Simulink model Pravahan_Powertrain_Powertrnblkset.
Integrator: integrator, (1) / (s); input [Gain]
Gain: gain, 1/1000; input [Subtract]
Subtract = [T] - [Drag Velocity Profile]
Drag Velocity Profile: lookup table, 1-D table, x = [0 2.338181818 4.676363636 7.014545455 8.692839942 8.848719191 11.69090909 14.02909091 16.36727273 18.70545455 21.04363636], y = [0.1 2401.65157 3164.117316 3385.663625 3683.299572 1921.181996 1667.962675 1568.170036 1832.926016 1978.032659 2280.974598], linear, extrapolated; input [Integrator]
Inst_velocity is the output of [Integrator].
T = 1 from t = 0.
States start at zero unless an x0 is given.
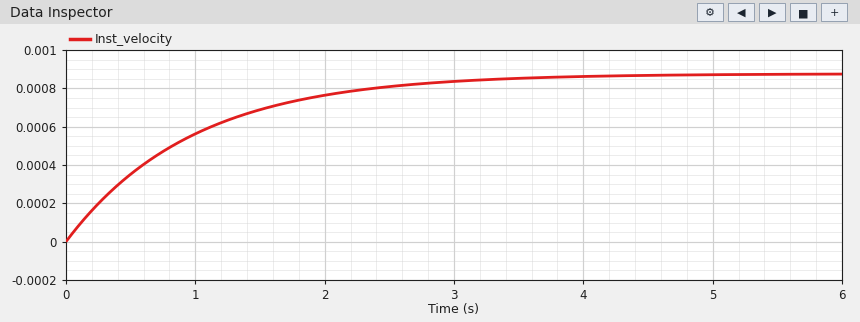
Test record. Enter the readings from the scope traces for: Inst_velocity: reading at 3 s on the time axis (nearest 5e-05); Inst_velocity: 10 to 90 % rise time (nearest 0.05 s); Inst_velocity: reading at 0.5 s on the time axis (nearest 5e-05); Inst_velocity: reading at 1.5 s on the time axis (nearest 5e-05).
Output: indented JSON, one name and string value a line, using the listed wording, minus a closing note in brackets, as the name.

{
  "Inst_velocity: reading at 3 s on the time axis": "0.00085",
  "Inst_velocity: 10 to 90 % rise time": "2.15 s",
  "Inst_velocity: reading at 0.5 s on the time axis": "0.00035",
  "Inst_velocity: reading at 1.5 s on the time axis": "0.00070"
}
